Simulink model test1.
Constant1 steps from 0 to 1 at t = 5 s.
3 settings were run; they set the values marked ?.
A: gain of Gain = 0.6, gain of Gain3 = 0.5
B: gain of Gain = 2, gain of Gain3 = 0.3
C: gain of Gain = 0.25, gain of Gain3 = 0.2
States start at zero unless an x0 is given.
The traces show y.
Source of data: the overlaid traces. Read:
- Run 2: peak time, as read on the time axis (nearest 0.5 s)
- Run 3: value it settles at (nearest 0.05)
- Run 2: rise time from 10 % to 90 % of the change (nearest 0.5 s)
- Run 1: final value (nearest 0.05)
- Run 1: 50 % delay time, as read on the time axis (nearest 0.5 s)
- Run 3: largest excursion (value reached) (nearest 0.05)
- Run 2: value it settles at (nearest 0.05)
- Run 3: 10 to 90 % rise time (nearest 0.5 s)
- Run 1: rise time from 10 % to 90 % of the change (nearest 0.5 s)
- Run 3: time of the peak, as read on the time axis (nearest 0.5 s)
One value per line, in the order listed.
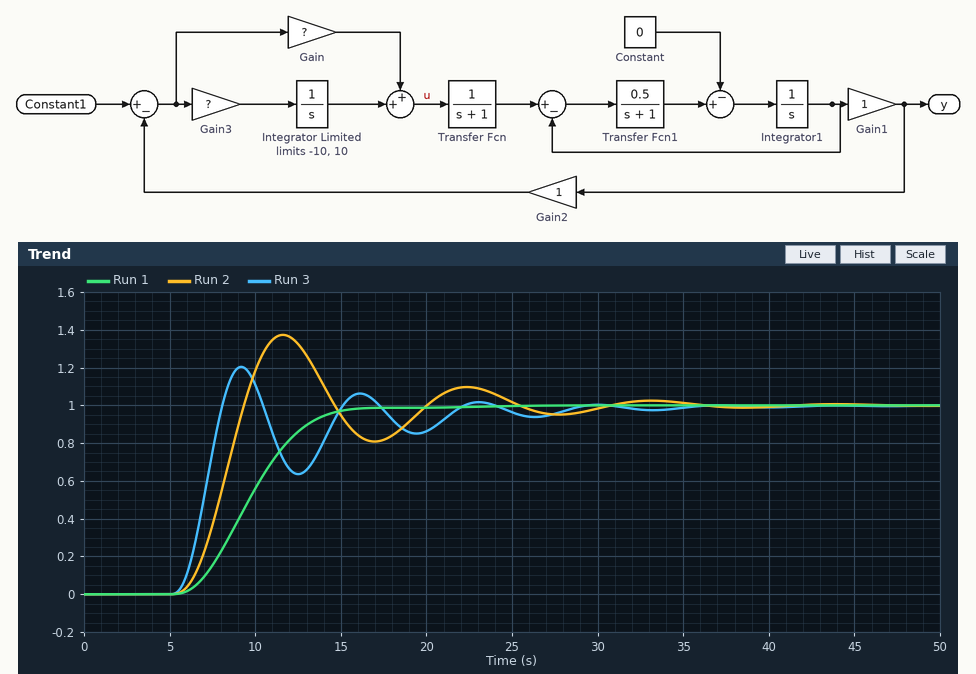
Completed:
11.5 s
1.00
2.5 s
1.00
9.5 s
1.20
1.00
2.0 s
6.0 s
9.0 s
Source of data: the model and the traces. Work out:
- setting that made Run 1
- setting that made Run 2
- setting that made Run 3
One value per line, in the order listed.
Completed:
C
A
B
